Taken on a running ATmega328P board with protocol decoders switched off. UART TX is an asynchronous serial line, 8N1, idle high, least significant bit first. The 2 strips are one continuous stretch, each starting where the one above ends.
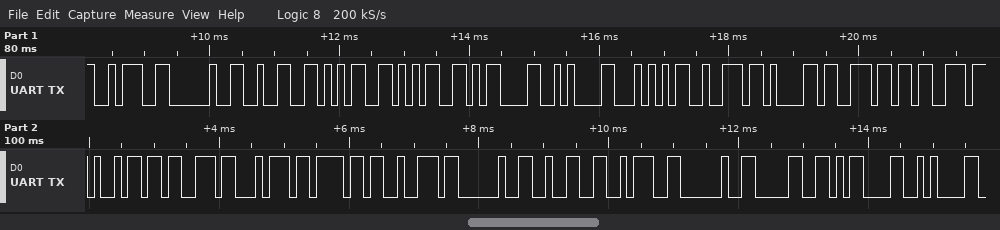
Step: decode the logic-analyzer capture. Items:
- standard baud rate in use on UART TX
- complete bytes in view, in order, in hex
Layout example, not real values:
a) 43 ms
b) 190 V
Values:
a) 9600 baud
b) 3A 20 32 35 35 0D 0A 54 72 61 6E 73 69 73 74 6F 72 20 32 3A 20 30 0D 0A
